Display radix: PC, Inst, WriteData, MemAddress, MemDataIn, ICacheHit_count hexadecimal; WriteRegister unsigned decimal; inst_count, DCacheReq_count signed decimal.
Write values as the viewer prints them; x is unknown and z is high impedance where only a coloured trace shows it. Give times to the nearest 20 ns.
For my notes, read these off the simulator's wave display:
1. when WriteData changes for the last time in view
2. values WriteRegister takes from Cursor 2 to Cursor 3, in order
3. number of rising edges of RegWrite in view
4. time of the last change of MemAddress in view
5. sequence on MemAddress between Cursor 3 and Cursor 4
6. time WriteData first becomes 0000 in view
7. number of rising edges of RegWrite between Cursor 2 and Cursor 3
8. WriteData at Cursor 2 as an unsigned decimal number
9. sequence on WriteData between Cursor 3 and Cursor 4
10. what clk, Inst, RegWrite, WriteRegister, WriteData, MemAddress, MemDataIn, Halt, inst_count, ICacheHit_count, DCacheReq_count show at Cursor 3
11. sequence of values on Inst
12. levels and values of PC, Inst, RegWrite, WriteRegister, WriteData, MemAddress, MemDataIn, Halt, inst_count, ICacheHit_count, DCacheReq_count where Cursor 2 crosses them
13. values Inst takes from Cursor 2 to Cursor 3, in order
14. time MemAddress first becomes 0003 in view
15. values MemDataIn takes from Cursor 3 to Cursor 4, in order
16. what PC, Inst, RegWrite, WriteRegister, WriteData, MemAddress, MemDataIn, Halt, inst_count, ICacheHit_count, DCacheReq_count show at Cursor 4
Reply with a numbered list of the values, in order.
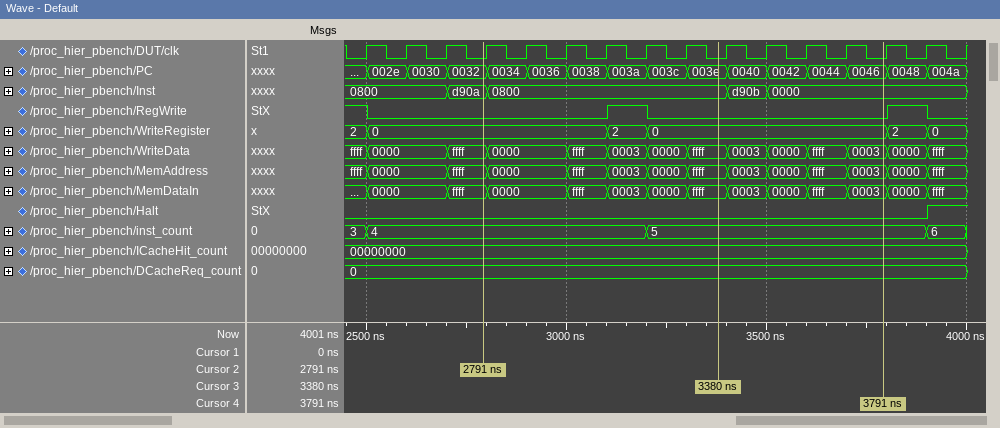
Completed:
1. 3900 ns
2. 0, 2, 0
3. 2
4. 3900 ns
5. ffff, 0003, 0000, ffff, 0003
6. 2500 ns
7. 1
8. 65535
9. ffff, 0003, 0000, ffff, 0003
10. clk=0, Inst=0800, RegWrite=0, WriteRegister=0, WriteData=ffff, MemAddress=ffff, MemDataIn=ffff, Halt=0, inst_count=5, ICacheHit_count=00000000, DCacheReq_count=0
11. 0800, d90a, 0800, d90b, 0000
12. PC=0032, Inst=d90a, RegWrite=0, WriteRegister=0, WriteData=ffff, MemAddress=ffff, MemDataIn=ffff, Halt=0, inst_count=4, ICacheHit_count=00000000, DCacheReq_count=0
13. d90a, 0800
14. 3100 ns
15. ffff, 0003, 0000, ffff, 0003
16. PC=0046, Inst=0000, RegWrite=0, WriteRegister=0, WriteData=0003, MemAddress=0003, MemDataIn=0003, Halt=0, inst_count=5, ICacheHit_count=00000000, DCacheReq_count=0
